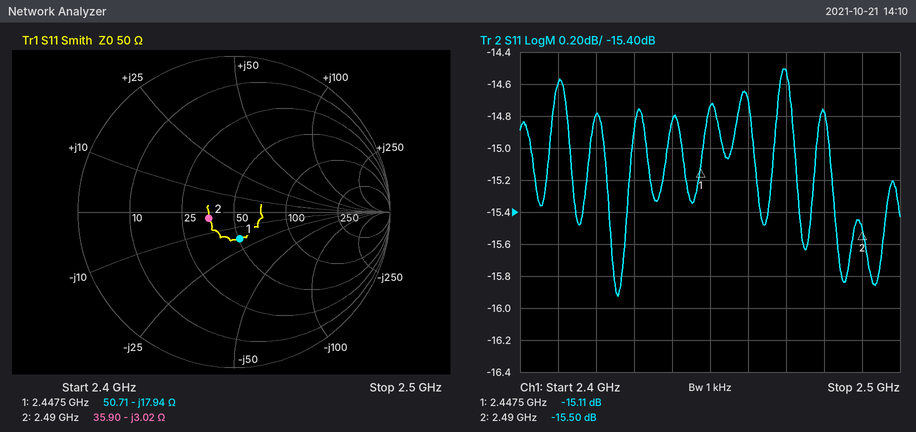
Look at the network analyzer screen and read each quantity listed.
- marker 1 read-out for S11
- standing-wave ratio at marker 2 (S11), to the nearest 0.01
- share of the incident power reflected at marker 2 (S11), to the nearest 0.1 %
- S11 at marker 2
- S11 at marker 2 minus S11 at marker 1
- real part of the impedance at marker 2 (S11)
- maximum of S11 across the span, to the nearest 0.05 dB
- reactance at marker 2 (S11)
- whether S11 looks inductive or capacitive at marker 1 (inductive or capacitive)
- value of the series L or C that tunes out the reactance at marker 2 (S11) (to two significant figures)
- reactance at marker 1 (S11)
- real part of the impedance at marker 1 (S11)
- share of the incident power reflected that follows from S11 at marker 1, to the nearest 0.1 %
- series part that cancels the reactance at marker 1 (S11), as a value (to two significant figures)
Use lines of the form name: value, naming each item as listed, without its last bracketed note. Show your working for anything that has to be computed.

marker 1 read-out for S11: -15.11 dB
standing-wave ratio at marker 2 (S11), to the nearest 0.01: 1.40
share of the incident power reflected at marker 2 (S11), to the nearest 0.1 %: 10^(-15.5/10) ≈ 2.8 %
S11 at marker 2: -15.50 dB
S11 at marker 2 minus S11 at marker 1: -15.5 − (-15.11) = -0.39 dB
real part of the impedance at marker 2: 35.90 Ω
maximum of S11 across the span, to the nearest 0.05 dB: -14.50 dB
reactance at marker 2: -3.02 Ω
whether S11 looks inductive or capacitive at marker 1: capacitive
value of the series L or C that tunes out the reactance at marker 2 (S11): L = 3.02 Ω/(2π × 2.49 GHz) ≈ 193 pH, so 190 pH to two significant figures
reactance at marker 1: -17.94 Ω
real part of the impedance at marker 1: 50.71 Ω
share of the incident power reflected that follows from S11 at marker 1, to the nearest 0.1 %: 10^(-15.11/10) ≈ 3.1 %
series part that cancels the reactance at marker 1 (S11), as a value: L = 17.94 Ω/(2π × 2.4475 GHz) ≈ 1.2 nH
